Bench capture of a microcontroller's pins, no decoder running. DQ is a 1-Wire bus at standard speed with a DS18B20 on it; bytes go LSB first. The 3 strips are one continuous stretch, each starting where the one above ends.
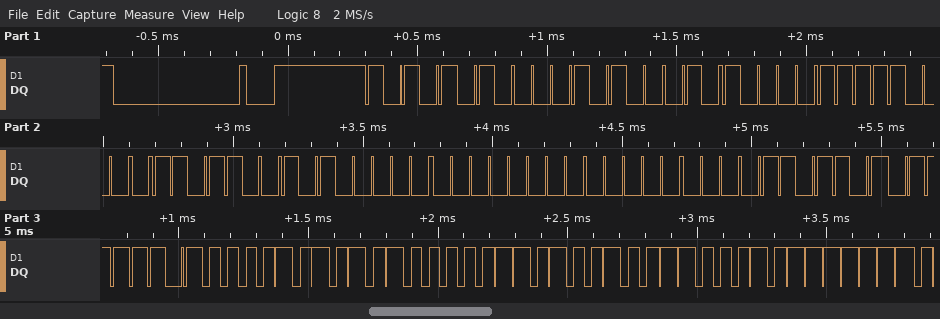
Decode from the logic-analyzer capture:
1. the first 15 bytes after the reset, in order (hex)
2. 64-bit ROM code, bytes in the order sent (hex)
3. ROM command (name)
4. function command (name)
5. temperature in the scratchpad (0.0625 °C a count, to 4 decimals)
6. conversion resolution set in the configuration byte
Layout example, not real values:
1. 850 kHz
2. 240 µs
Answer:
1. 55 28 0A 1F 36 05 00 00 B6 BE 50 05 4B 46 7F
2. 28 0A 1F 36 05 00 00 B6
3. Match ROM
4. Read Scratchpad
5. 85.0000 °C
6. 12 bits
